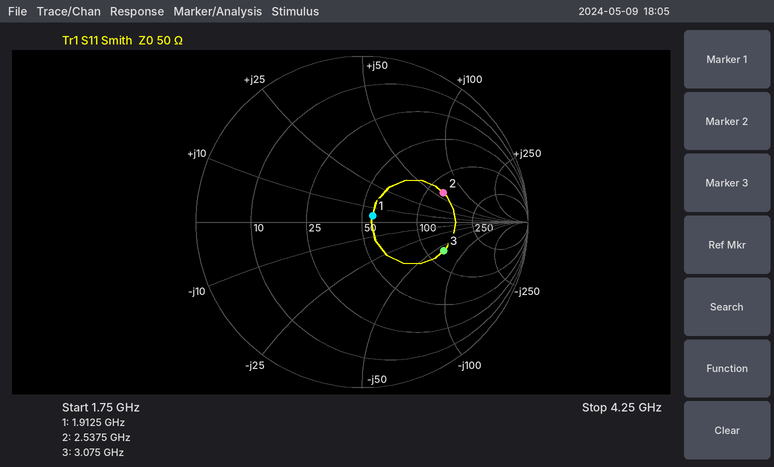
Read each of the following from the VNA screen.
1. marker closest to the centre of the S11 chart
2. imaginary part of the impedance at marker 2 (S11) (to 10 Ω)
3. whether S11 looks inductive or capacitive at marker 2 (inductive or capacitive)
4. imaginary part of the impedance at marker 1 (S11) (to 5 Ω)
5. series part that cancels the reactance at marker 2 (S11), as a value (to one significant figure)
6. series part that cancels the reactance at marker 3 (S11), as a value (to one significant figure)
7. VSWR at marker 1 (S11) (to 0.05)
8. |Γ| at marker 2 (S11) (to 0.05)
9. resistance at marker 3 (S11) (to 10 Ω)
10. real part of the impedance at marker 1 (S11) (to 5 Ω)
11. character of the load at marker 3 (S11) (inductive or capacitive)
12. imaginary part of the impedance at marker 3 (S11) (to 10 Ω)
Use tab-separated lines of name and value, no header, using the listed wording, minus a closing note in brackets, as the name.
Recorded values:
marker closest to the centre of the S11 chart	marker 1
imaginary part of the impedance at marker 2 (S11)	+60 Ω
whether S11 looks inductive or capacitive at marker 2	inductive
imaginary part of the impedance at marker 1 (S11)	+5 Ω
series part that cancels the reactance at marker 2 (S11), as a value	1 pF
series part that cancels the reactance at marker 3 (S11), as a value	3 nH
VSWR at marker 1 (S11)	1.15
|Γ| at marker 2 (S11)	0.50
resistance at marker 3 (S11)	130 Ω
real part of the impedance at marker 1 (S11)	55 Ω
character of the load at marker 3 (S11)	capacitive
imaginary part of the impedance at marker 3 (S11)	-60 Ω
